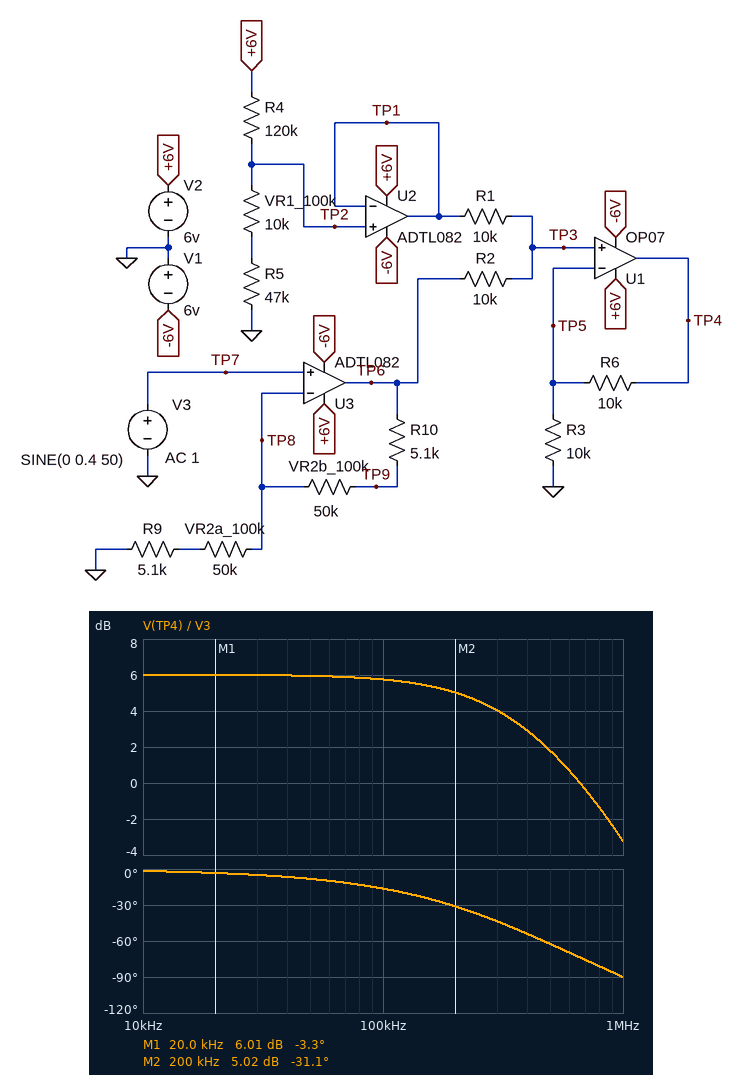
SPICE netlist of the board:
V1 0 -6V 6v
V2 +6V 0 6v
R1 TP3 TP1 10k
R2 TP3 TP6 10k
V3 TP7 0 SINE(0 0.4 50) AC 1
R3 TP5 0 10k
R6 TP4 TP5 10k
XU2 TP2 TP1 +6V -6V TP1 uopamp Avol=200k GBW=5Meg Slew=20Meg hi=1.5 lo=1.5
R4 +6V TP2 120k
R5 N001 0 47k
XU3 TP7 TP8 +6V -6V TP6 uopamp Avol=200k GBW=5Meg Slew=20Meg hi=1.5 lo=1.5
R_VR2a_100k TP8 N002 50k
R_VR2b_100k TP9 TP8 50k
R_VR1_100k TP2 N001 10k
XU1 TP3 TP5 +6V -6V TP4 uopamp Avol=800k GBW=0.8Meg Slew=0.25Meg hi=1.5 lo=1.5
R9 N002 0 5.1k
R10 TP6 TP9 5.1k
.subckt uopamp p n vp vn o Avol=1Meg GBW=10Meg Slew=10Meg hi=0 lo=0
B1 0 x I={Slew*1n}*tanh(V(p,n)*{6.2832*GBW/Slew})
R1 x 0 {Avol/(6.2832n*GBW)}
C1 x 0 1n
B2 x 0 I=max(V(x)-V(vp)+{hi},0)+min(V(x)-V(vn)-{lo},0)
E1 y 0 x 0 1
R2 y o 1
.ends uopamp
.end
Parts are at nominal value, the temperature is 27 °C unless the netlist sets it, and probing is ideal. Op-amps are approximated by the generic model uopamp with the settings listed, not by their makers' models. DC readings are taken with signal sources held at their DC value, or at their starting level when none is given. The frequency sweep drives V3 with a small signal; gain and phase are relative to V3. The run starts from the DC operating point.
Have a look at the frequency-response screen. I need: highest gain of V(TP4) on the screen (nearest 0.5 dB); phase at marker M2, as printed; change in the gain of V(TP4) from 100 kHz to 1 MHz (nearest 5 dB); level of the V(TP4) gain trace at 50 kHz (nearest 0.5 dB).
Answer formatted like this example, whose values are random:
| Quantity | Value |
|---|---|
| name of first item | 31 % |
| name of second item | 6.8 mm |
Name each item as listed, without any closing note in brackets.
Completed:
| Quantity | Value |
|---|---|
| highest gain of V(TP4) on the screen | 6.0 dB |
| phase at marker M2, as printed | -31.1 deg |
| change in the gain of V(TP4) from 100 kHz to 1 MHz | -10 dB |
| level of the V(TP4) gain trace at 50 kHz | 6.0 dB |
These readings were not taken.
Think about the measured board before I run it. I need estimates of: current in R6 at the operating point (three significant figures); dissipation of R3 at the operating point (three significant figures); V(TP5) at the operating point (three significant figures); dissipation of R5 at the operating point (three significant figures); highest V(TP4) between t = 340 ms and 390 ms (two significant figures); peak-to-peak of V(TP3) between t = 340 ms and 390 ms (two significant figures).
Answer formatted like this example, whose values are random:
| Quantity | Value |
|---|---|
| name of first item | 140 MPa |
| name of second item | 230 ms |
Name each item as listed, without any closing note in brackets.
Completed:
| Quantity | Value |
|---|---|
| current in R6 at the operating point | 96.6 µA |
| dissipation of R3 at the operating point | 93.3 µW |
| V(TP5) at the operating point | 966 mV |
| dissipation of R5 at the operating point | 54.0 µW |
| highest V(TP4) between t = 340 ms and 390 ms | 2.7 V |
| peak-to-peak of V(TP3) between t = 340 ms and 390 ms | 800 mV |
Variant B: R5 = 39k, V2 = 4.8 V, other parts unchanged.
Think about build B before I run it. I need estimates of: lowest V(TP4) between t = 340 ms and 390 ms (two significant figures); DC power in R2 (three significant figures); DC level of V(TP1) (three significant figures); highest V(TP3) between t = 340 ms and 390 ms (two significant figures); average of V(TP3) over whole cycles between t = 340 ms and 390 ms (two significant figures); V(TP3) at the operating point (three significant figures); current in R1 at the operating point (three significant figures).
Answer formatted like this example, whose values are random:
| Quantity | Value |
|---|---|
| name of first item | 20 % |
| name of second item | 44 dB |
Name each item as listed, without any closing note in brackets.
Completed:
| Quantity | Value |
|---|---|
| lowest V(TP4) between t = 340 ms and 390 ms | 590 mV |
| DC power in R2 | 48.4 µW |
| DC level of V(TP1) | 1.39 V |
| highest V(TP3) between t = 340 ms and 390 ms | 1.1 V |
| average of V(TP3) over whole cycles between t = 340 ms and 390 ms | 700 mV |
| V(TP3) at the operating point | 696 mV |
| current in R1 at the operating point | 69.6 µA |
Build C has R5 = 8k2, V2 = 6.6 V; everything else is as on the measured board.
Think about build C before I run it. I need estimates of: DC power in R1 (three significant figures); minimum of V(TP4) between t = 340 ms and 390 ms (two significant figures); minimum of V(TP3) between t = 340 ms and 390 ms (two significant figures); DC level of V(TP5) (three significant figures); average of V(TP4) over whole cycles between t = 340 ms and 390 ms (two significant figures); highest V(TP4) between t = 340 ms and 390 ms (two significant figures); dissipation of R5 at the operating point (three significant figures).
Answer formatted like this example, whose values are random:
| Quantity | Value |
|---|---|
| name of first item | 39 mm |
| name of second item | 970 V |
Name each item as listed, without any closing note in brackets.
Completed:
| Quantity | Value |
|---|---|
| DC power in R1 | 18.9 µW |
| minimum of V(TP4) between t = 340 ms and 390 ms | 69 mV |
| minimum of V(TP3) between t = 340 ms and 390 ms | 35 mV |
| DC level of V(TP5) | 435 mV |
| average of V(TP4) over whole cycles between t = 340 ms and 390 ms | 870 mV |
| highest V(TP4) between t = 340 ms and 390 ms | 1.7 V |
| dissipation of R5 at the operating point | 18.7 µW |
